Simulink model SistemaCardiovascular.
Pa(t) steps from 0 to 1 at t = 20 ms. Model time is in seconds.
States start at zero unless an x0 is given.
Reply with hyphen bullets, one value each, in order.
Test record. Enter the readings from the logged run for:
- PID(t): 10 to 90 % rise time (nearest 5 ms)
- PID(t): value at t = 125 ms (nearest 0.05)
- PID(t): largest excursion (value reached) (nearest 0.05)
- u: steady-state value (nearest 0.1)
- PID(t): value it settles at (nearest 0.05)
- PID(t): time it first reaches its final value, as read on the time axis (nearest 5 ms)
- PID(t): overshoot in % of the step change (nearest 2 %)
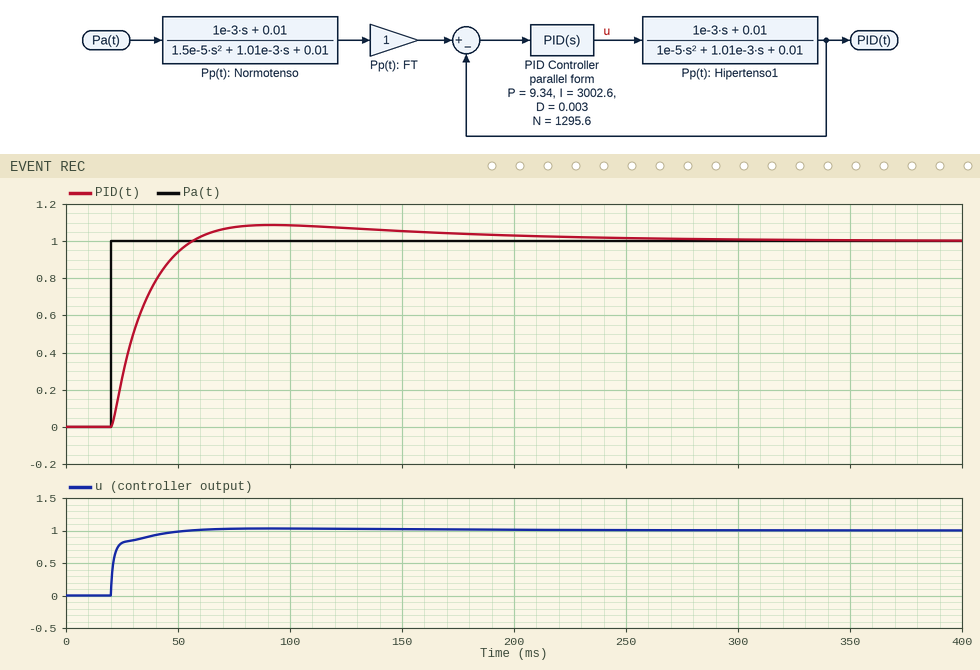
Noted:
- 25 ms
- 1.05
- 1.10
- 1.0
- 1.00
- 55 ms
- 8 %
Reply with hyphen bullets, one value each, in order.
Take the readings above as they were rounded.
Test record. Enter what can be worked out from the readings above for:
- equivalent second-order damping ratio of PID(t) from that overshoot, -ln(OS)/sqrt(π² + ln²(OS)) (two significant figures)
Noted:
- 0.63
